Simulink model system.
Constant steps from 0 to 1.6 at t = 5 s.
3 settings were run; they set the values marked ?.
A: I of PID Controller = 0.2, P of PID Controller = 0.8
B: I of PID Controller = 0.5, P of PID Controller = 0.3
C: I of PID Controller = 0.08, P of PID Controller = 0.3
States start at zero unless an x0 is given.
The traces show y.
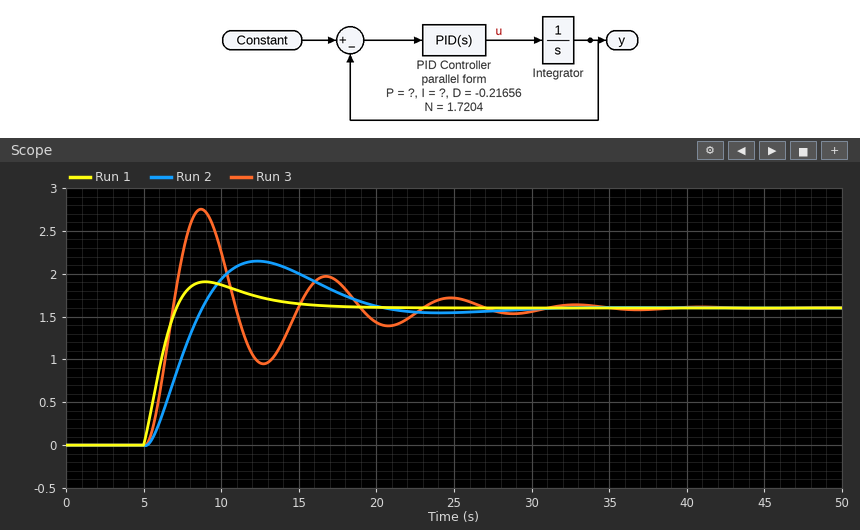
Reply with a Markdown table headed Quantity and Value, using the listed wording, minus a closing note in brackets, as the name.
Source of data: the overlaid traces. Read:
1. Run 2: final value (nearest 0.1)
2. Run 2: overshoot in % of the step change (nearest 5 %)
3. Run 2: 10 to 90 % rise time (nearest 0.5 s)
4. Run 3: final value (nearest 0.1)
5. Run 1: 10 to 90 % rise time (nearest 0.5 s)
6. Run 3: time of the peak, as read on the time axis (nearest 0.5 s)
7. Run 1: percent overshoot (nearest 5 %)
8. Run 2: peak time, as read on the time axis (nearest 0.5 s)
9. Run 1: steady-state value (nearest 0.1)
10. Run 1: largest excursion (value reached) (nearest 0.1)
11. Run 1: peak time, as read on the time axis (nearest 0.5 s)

| Quantity | Value |
|---|---|
| Run 2: final value | 1.6 |
| Run 2: overshoot in % of the step change | 35 % |
| Run 2: 10 to 90 % rise time | 2.5 s |
| Run 3: final value | 1.6 |
| Run 1: 10 to 90 % rise time | 1.5 s |
| Run 3: time of the peak, as read on the time axis | 8.5 s |
| Run 1: percent overshoot | 20 % |
| Run 2: peak time, as read on the time axis | 12.5 s |
| Run 1: steady-state value | 1.6 |
| Run 1: largest excursion (value reached) | 1.9 |
| Run 1: peak time, as read on the time axis | 9.0 s |
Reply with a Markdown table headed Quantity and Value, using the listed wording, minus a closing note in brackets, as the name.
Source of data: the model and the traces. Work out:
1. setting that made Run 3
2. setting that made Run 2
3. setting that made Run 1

| Quantity | Value |
|---|---|
| setting that made Run 3 | B |
| setting that made Run 2 | C |
| setting that made Run 1 | A |
